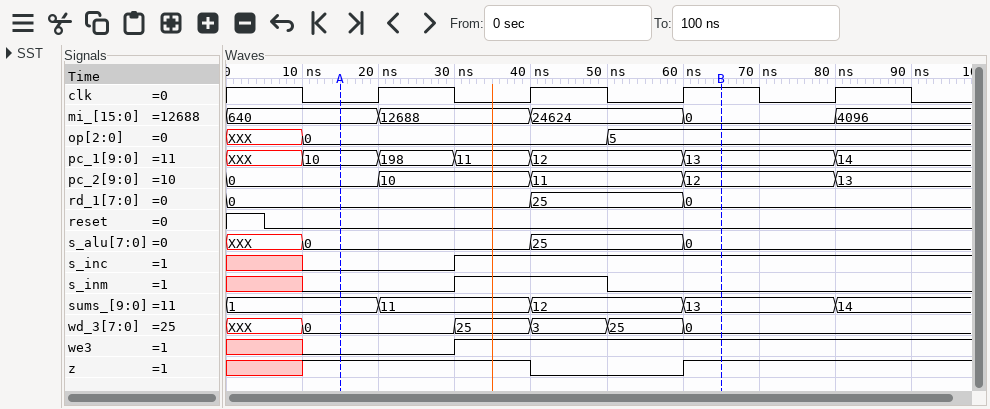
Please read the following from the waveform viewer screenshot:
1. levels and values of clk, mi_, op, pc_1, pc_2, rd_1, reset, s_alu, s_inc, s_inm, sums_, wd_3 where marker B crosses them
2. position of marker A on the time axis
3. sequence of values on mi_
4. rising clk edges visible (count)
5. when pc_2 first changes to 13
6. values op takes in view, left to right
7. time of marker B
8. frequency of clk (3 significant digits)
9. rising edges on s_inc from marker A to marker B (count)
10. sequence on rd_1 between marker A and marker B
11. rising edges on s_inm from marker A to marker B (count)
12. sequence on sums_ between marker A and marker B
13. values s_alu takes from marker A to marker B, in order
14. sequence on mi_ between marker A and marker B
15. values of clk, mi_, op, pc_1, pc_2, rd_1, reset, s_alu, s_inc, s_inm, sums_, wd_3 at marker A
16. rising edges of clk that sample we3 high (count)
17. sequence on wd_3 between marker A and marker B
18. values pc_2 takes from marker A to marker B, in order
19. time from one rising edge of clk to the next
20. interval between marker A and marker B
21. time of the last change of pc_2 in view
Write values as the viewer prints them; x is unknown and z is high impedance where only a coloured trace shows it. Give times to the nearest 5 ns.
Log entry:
clk=1, mi_=0, op=5, pc_1=13, pc_2=12, rd_1=0, reset=0, s_alu=0, s_inc=1, s_inm=0, sums_=13, wd_3=0
15 ns
640, 12688, 24624, 0, 4096
4
80 ns
XXX, 0, 5
65 ns
50.0 MHz
1
0, 25, 0
1
1, 11, 12, 13
0, 25, 0
640, 12688, 24624, 0
clk=0, mi_=640, op=0, pc_1=10, pc_2=0, rd_1=0, reset=0, s_alu=0, s_inc=0, s_inm=0, sums_=1, wd_3=0
3
0, 25, 3, 25, 0
0, 10, 11, 12
20 ns
50 ns
80 ns
